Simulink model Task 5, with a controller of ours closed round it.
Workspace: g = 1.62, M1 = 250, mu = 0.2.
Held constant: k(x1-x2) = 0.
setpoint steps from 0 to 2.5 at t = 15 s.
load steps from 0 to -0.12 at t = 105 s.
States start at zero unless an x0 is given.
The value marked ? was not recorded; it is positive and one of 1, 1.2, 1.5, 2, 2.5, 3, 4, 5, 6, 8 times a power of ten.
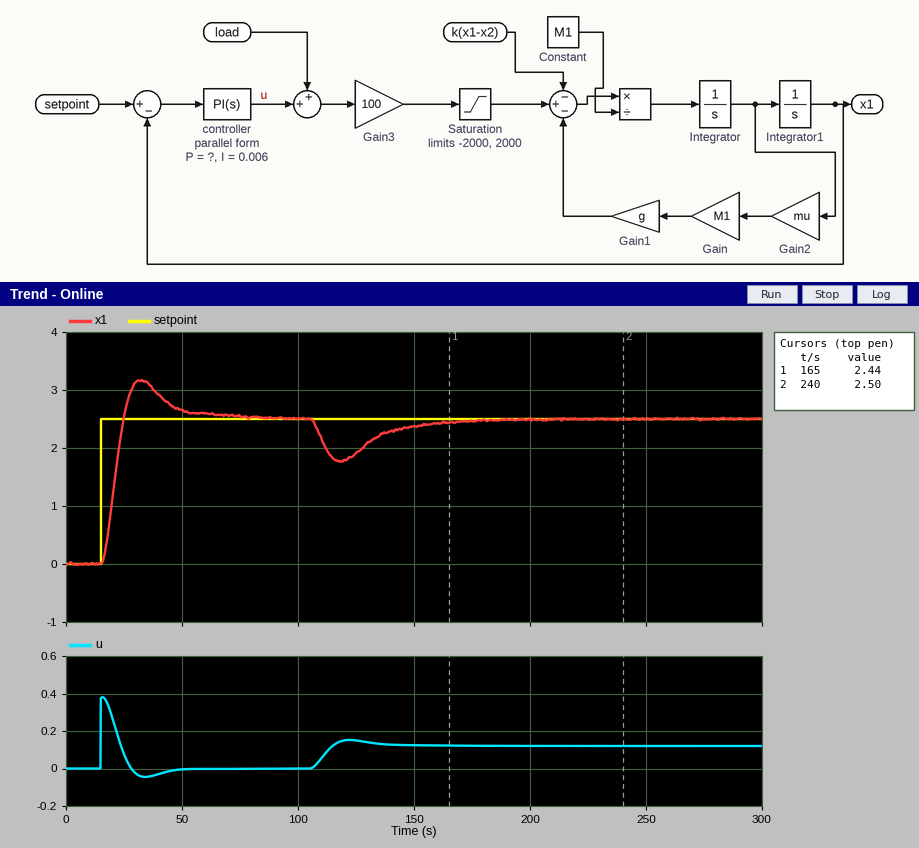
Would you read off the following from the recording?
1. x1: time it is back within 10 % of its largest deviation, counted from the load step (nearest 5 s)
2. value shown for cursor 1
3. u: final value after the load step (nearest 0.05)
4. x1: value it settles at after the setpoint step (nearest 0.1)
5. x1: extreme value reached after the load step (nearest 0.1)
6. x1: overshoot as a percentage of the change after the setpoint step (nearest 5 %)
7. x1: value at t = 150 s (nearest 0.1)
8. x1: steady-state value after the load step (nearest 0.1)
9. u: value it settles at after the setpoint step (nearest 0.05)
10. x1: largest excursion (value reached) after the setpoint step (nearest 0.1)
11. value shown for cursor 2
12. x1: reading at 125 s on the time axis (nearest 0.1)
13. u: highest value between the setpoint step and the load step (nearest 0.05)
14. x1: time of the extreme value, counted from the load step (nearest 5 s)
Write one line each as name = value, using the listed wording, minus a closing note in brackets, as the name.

x1: time it is back within 10 % of its largest deviation, counted from the load step = 55 s
value shown for cursor 1 = 2.44
u: final value after the load step = 0.10
x1: value it settles at after the setpoint step = 2.5
x1: extreme value reached after the load step = 1.8
x1: overshoot as a percentage of the change after the setpoint step = 25 %
x1: value at t = 150 s = 2.4
x1: steady-state value after the load step = 2.5
u: value it settles at after the setpoint step = 0.00
x1: largest excursion (value reached) after the setpoint step = 3.2
value shown for cursor 2 = 2.50
x1: reading at 125 s on the time axis = 1.9
u: highest value between the setpoint step and the load step = 0.40
x1: time of the extreme value, counted from the load step = 15 s
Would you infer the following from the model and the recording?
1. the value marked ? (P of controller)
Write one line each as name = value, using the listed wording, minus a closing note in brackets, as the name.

the value marked ? = 0.15
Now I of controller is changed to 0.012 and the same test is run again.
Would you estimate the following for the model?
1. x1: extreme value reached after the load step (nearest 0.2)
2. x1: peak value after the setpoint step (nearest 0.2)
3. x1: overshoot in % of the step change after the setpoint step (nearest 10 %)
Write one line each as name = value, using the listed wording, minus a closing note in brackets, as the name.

x1: extreme value reached after the load step = 1.8
x1: peak value after the setpoint step = 3.6
x1: overshoot in % of the step change after the setpoint step = 40 %
